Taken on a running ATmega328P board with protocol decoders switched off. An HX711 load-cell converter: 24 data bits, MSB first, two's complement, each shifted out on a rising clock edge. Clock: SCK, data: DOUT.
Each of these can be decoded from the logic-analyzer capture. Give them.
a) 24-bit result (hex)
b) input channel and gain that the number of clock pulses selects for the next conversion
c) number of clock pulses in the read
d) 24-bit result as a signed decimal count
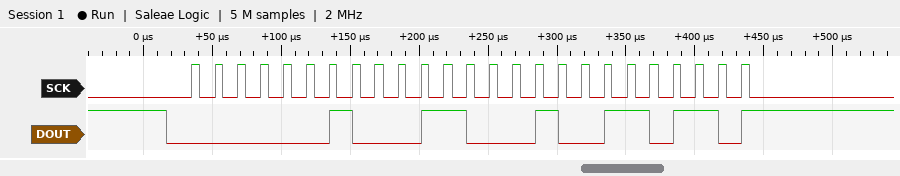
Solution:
0x023136
channel A, gain 128
25
143670
